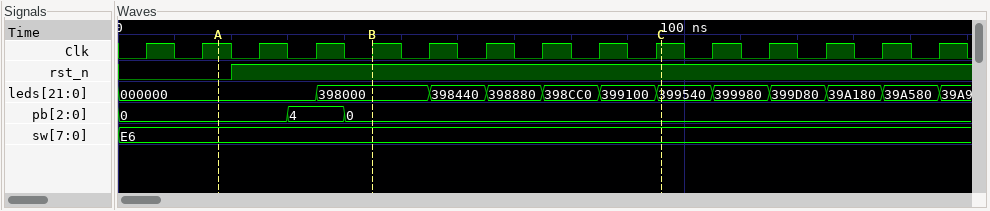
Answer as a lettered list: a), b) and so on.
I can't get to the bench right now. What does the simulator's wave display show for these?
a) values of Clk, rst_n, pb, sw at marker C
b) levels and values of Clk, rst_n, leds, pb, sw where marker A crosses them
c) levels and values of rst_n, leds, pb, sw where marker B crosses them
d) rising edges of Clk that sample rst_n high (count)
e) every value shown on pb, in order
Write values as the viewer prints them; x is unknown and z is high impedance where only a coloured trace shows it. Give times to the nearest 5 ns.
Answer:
a) Clk=1, rst_n=1, pb=0, sw=E6
b) Clk=1, rst_n=0, leds=000000, pb=0, sw=E6
c) rst_n=1, leds=398000, pb=0, sw=E6
d) 13
e) 0, 4, 0
